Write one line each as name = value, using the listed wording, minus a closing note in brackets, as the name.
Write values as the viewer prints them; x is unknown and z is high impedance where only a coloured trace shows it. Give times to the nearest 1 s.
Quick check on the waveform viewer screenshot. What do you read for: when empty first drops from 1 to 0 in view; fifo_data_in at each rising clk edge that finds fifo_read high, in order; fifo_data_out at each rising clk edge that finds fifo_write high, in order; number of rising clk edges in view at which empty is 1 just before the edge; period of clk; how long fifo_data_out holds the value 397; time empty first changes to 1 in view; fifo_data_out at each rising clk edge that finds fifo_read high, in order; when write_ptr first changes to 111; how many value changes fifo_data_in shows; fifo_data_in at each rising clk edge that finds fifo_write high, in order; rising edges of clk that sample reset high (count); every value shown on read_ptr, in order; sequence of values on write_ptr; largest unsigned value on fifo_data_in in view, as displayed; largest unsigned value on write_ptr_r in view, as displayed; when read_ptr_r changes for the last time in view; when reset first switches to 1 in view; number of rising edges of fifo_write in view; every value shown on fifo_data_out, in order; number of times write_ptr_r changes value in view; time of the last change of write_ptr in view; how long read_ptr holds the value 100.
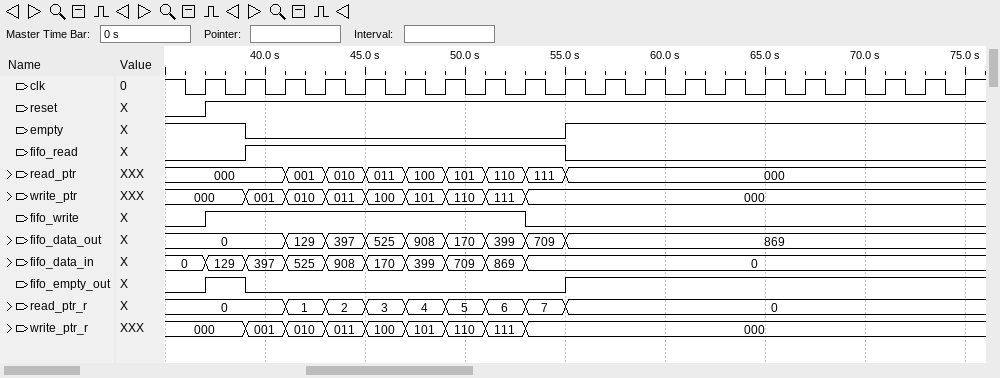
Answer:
when empty first drops from 1 to 0 in view = 39 s
fifo_data_in at each rising clk edge that finds fifo_read high, in order = 397, 525, 908, 170, 399, 709, 869, 0
fifo_data_out at each rising clk edge that finds fifo_write high, in order = 0, 0, 129, 397, 525, 908, 170, 399
number of rising clk edges in view at which empty is 1 just before the edge = 12
period of clk = 2 s
how long fifo_data_out holds the value 397 = 2 s
time empty first changes to 1 in view = 55 s
fifo_data_out at each rising clk edge that finds fifo_read high, in order = 0, 129, 397, 525, 908, 170, 399, 709
when write_ptr first changes to 111 = 51 s
how many value changes fifo_data_in shows = 9
fifo_data_in at each rising clk edge that finds fifo_write high, in order = 129, 397, 525, 908, 170, 399, 709, 869
rising edges of clk that sample reset high = 19
every value shown on read_ptr, in order = 000, 001, 010, 011, 100, 101, 110, 111, 000
sequence of values on write_ptr = 000, 001, 010, 011, 100, 101, 110, 111, 000
largest unsigned value on fifo_data_in in view, as displayed = 908
largest unsigned value on write_ptr_r in view, as displayed = 111
when read_ptr_r changes for the last time in view = 55 s
when reset first switches to 1 in view = 37 s
number of rising edges of fifo_write in view = 1
every value shown on fifo_data_out, in order = 0, 129, 397, 525, 908, 170, 399, 709, 869
number of times write_ptr_r changes value in view = 8
time of the last change of write_ptr in view = 53 s
how long read_ptr holds the value 100 = 2 s
